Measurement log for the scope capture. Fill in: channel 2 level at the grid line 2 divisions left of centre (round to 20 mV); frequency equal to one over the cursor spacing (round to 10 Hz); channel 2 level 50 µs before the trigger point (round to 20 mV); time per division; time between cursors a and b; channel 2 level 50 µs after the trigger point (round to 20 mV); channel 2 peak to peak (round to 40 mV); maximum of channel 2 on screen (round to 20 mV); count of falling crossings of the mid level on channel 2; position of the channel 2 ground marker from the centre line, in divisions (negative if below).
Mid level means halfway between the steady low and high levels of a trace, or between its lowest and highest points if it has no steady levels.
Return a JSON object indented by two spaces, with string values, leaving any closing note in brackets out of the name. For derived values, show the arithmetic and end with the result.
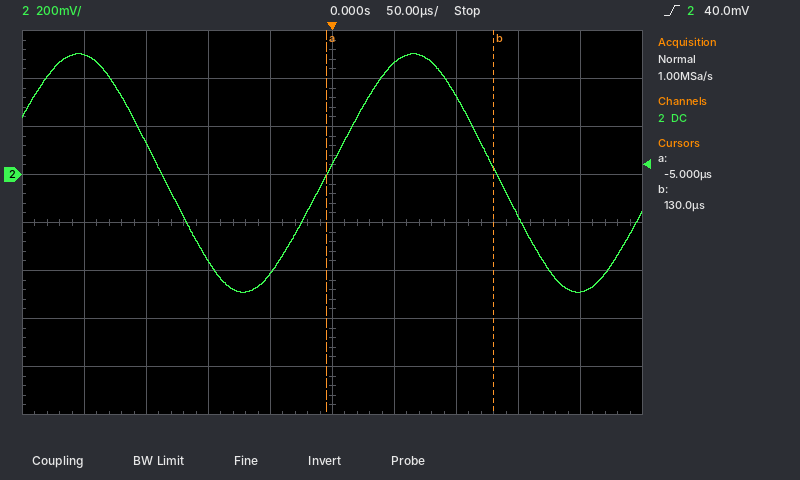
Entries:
{
  "channel 2 level at the grid line 2 divisions left of centre": "-360 mV",
  "frequency equal to one over the cursor spacing": "1 / 135 µs ≈ 7.41 kHz",
  "channel 2 level 50 µs before the trigger point": "-420 mV",
  "time per division": "50 µs",
  "time between cursors a and b": "130 µs − (-5 µs) = 135 µs",
  "channel 2 level 50 µs after the trigger point": "460 mV",
  "channel 2 peak to peak": "1.00 V",
  "maximum of channel 2 on screen": "500 mV",
  "count of falling crossings of the mid level on channel 2": "2",
  "position of the channel 2 ground marker from the centre line, in divisions": "+1.0 div"
}
